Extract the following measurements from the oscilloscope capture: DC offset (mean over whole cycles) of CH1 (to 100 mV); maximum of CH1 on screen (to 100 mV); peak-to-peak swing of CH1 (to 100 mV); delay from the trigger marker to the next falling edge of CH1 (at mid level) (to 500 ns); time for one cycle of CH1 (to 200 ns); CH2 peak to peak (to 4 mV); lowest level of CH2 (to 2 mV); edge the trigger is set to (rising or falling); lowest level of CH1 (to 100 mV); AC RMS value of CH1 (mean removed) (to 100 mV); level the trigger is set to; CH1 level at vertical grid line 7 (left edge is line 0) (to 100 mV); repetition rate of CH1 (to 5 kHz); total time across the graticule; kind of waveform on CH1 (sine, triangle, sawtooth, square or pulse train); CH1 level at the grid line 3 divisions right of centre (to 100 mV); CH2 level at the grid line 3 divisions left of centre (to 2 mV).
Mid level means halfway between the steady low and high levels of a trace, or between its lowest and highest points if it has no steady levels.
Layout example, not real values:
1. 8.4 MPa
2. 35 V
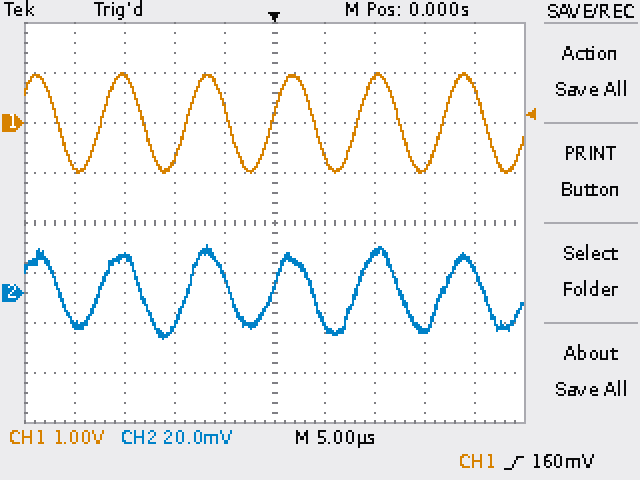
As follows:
1. 0.0 V
2. 1.0 V
3. 2.0 V
4. 4.0 µs
5. 8.6 µs
6. 36 mV
7. -18 mV
8. rising
9. -1.0 V
10. 700 mV
11. 160 mV
12. 900 mV
13. 115 kHz
14. 50 µs
15. sine
16. -900 mV
17. 14 mV
